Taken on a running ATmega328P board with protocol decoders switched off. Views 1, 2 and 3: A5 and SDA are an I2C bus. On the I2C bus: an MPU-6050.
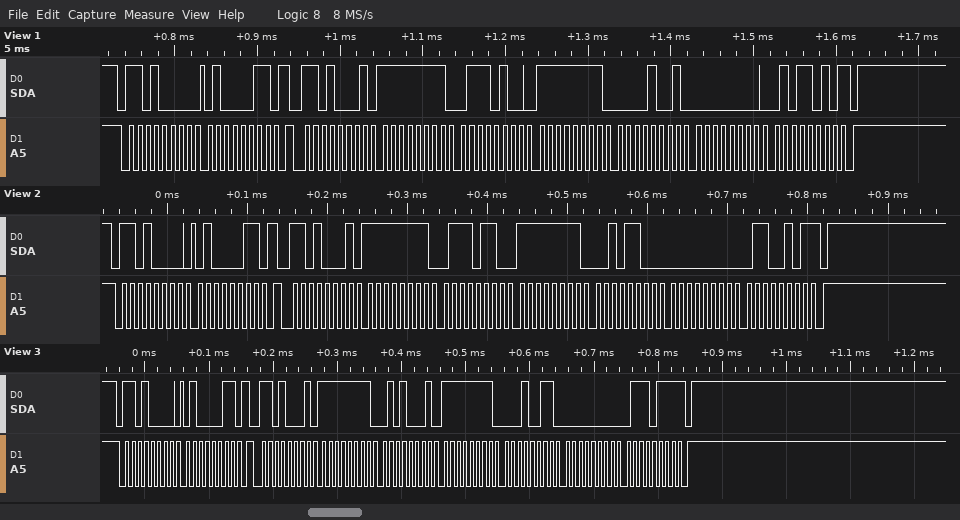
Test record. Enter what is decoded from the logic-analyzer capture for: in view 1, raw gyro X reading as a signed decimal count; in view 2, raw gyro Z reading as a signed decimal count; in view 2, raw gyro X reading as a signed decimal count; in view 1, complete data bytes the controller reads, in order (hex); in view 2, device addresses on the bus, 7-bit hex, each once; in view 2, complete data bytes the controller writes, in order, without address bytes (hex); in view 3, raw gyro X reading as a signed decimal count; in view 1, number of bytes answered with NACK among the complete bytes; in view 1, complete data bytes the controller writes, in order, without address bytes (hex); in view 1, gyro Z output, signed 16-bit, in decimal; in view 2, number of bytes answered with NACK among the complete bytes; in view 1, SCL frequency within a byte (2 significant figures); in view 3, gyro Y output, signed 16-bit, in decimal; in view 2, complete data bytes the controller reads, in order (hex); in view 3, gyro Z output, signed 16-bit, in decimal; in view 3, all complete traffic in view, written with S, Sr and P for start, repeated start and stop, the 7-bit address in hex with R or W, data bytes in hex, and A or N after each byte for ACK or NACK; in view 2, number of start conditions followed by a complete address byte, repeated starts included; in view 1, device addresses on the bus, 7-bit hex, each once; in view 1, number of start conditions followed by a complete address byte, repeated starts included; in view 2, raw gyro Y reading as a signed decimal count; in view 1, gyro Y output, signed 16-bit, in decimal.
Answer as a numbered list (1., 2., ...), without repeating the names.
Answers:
1. -140
2. 101
3. -138
4. FF 74 FF 09 00 5A
5. 0x68
6. 43
7. -175
8. 1
9. 43
10. 90
11. 1
12. 100 kHz
13. -237
14. FF 76 FF 2C 00 65
15. 119
16. S 68W A 43 A Sr 68R A FF A 51 A FF A 13 A 00 A 77 N P
17. 2
18. 0x68
19. 2
20. -212
21. -247
